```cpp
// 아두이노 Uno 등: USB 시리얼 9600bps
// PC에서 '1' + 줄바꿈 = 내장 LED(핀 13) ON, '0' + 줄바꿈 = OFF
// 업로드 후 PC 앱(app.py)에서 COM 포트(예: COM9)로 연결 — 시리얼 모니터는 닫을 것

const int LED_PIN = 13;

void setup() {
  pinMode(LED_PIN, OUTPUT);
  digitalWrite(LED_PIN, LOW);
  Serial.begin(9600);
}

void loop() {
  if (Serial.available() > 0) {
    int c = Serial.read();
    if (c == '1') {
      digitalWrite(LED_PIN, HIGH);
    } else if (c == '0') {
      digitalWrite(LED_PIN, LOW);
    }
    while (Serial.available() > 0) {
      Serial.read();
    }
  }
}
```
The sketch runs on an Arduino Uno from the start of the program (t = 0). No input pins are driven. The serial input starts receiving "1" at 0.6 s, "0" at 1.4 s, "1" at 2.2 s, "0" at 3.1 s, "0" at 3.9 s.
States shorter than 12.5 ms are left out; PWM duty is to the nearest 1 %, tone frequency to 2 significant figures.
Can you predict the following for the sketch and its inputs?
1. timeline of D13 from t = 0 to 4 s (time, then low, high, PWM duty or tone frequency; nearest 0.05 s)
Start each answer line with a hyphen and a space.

- 0 s low; 0.6 s high; 1.4 s low; 2.2 s high; 3.1 s low
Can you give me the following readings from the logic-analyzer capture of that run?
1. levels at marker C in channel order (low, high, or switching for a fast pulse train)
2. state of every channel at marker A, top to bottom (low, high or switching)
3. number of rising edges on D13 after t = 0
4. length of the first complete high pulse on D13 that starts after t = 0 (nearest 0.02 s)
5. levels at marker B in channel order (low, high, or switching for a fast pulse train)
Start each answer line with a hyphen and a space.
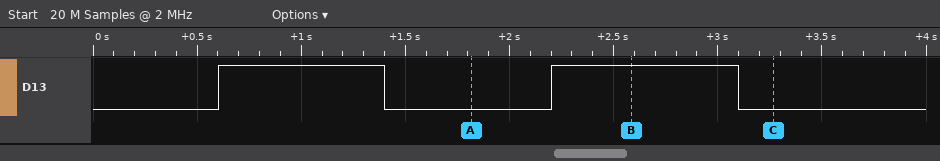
- D13 low
- D13 low
- 2
- 0.80 s
- D13 high
